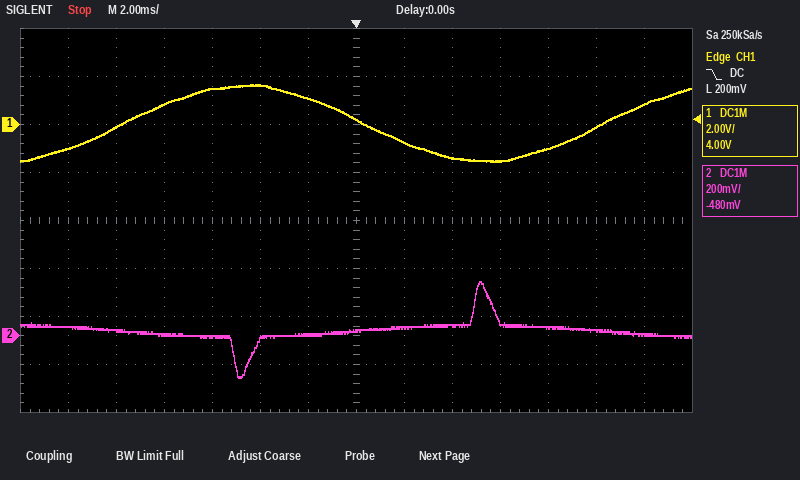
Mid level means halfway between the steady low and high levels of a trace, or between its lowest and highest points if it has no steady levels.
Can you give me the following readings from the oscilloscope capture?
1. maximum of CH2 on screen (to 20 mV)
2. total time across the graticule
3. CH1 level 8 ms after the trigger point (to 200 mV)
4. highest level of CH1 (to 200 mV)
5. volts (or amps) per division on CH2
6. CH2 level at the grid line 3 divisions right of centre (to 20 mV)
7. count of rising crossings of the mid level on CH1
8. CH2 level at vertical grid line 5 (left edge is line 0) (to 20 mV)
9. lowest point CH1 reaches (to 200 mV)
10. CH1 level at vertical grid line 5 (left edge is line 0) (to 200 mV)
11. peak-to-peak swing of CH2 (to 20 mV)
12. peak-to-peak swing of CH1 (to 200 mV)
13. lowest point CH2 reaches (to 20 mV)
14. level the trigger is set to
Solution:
220 mV
28 ms
-1.0 V
1.6 V
200 mV
60 mV
2
-20 mV
-1.6 V
1.6 V
400 mV
3.2 V
-180 mV
200 mV
